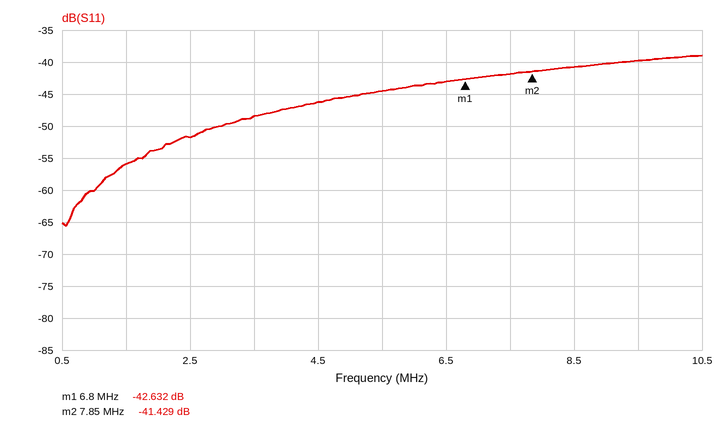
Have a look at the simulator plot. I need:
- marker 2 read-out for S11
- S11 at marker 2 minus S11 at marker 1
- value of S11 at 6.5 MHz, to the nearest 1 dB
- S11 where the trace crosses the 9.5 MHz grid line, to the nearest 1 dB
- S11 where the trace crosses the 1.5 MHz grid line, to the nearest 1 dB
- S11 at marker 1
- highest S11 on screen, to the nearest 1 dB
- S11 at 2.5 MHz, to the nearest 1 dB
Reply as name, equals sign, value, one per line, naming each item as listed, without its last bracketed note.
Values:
marker 2 read-out for S11 = -41.429 dB
S11 at marker 2 minus S11 at marker 1 = 1.203 dB
value of S11 at 6.5 MHz, to the nearest 1 dB = -43 dB
S11 where the trace crosses the 9.5 MHz grid line, to the nearest 1 dB = -40 dB
S11 where the trace crosses the 1.5 MHz grid line, to the nearest 1 dB = -56 dB
S11 at marker 1 = -42.632 dB
highest S11 on screen, to the nearest 1 dB = -39 dB
S11 at 2.5 MHz, to the nearest 1 dB = -52 dB
